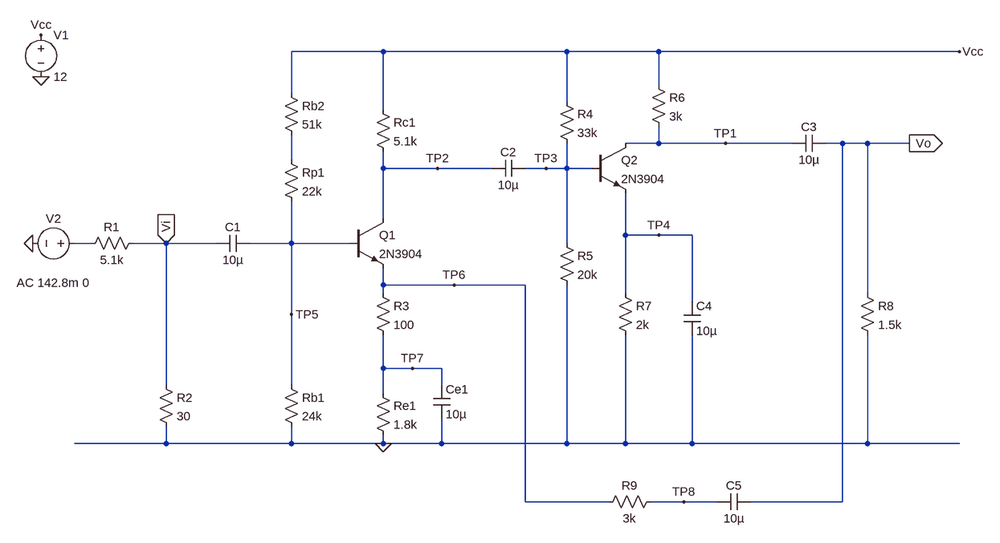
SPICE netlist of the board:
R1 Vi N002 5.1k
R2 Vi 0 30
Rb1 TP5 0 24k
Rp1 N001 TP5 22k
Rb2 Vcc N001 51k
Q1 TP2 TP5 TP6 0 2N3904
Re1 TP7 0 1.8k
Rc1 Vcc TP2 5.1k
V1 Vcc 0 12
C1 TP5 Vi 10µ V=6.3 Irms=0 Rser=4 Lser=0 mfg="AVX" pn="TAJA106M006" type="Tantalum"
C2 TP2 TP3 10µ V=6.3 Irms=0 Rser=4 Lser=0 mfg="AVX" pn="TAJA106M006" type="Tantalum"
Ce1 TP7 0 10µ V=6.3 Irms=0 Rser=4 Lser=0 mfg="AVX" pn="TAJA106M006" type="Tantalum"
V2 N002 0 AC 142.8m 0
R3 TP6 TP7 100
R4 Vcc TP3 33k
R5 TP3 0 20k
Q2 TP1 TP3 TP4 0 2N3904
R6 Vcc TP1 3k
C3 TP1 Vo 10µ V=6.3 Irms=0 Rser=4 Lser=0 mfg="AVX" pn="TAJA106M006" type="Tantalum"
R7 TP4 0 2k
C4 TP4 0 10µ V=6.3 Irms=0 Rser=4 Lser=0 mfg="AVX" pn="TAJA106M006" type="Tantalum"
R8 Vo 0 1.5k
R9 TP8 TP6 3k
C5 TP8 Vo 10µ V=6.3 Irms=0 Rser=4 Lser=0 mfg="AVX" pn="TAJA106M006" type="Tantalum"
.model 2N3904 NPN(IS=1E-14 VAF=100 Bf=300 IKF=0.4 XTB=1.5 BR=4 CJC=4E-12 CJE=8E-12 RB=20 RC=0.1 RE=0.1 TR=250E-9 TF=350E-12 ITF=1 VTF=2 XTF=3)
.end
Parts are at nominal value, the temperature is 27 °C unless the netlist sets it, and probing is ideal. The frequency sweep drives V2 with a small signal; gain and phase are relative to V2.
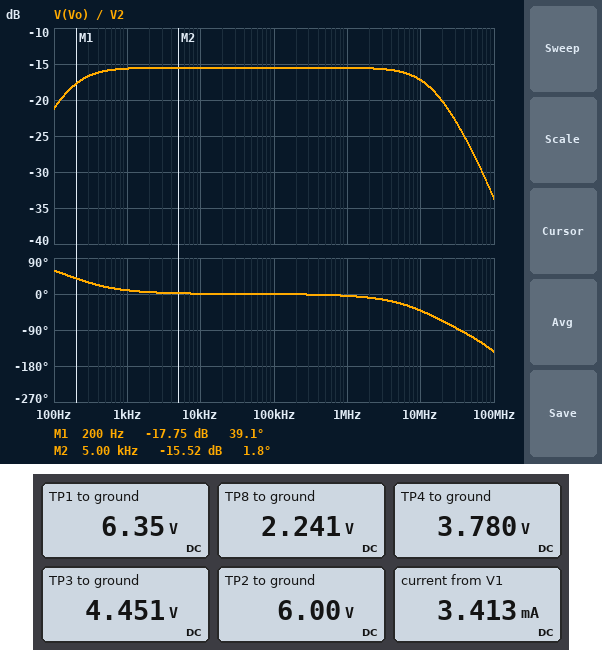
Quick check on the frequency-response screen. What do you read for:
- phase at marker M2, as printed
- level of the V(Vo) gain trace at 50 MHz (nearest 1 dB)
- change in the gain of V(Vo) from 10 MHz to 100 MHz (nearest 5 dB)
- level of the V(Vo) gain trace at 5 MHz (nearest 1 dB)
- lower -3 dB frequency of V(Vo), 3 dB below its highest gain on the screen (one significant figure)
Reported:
1.8 deg
-27 dB
-15 dB
-16 dB
200 Hz
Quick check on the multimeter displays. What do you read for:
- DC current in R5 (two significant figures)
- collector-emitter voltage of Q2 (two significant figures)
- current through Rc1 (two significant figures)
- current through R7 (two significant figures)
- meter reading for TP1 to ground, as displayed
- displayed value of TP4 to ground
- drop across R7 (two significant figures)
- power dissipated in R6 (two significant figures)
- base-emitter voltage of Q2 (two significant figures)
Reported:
220 µA
2.6 V
1.2 mA
1.9 mA
6.35 V
3.780 V
3.8 V
11 mW
670 mV
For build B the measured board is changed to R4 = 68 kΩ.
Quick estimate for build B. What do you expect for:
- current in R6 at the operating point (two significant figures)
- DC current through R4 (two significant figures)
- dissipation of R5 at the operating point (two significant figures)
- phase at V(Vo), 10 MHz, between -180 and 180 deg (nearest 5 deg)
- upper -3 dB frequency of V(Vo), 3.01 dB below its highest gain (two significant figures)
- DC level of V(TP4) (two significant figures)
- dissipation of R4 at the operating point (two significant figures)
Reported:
1.0 mA
140 µA
360 µW
-35 deg
17 MHz
2.0 V
1.3 mW
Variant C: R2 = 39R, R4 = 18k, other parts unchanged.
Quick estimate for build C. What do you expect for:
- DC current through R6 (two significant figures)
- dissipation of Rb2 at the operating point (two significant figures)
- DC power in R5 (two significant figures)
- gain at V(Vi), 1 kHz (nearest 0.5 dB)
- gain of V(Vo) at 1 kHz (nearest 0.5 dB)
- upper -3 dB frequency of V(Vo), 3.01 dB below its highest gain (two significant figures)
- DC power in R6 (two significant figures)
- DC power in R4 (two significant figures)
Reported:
2.4 mA
790 µW
1.5 mW
-42.5 dB
-35.5 dB
180 kHz
17 mW
2.3 mW
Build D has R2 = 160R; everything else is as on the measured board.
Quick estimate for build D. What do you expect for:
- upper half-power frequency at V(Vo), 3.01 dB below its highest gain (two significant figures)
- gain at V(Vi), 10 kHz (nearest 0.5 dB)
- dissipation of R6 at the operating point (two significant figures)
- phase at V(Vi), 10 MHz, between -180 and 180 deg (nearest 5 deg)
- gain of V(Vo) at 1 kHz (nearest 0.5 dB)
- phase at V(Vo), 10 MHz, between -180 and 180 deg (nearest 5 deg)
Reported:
15 MHz
-30.5 dB
11 mW
-5 deg
-1.5 dB
-45 deg
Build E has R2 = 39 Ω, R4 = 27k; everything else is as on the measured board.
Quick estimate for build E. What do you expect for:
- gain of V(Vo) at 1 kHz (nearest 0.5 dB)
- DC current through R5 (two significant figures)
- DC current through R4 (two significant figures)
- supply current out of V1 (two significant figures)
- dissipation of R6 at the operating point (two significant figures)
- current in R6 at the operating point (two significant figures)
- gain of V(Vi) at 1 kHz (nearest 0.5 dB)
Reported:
-13.5 dB
250 µA
260 µA
3.7 mA
14 mW
2.2 mA
-42.5 dB
